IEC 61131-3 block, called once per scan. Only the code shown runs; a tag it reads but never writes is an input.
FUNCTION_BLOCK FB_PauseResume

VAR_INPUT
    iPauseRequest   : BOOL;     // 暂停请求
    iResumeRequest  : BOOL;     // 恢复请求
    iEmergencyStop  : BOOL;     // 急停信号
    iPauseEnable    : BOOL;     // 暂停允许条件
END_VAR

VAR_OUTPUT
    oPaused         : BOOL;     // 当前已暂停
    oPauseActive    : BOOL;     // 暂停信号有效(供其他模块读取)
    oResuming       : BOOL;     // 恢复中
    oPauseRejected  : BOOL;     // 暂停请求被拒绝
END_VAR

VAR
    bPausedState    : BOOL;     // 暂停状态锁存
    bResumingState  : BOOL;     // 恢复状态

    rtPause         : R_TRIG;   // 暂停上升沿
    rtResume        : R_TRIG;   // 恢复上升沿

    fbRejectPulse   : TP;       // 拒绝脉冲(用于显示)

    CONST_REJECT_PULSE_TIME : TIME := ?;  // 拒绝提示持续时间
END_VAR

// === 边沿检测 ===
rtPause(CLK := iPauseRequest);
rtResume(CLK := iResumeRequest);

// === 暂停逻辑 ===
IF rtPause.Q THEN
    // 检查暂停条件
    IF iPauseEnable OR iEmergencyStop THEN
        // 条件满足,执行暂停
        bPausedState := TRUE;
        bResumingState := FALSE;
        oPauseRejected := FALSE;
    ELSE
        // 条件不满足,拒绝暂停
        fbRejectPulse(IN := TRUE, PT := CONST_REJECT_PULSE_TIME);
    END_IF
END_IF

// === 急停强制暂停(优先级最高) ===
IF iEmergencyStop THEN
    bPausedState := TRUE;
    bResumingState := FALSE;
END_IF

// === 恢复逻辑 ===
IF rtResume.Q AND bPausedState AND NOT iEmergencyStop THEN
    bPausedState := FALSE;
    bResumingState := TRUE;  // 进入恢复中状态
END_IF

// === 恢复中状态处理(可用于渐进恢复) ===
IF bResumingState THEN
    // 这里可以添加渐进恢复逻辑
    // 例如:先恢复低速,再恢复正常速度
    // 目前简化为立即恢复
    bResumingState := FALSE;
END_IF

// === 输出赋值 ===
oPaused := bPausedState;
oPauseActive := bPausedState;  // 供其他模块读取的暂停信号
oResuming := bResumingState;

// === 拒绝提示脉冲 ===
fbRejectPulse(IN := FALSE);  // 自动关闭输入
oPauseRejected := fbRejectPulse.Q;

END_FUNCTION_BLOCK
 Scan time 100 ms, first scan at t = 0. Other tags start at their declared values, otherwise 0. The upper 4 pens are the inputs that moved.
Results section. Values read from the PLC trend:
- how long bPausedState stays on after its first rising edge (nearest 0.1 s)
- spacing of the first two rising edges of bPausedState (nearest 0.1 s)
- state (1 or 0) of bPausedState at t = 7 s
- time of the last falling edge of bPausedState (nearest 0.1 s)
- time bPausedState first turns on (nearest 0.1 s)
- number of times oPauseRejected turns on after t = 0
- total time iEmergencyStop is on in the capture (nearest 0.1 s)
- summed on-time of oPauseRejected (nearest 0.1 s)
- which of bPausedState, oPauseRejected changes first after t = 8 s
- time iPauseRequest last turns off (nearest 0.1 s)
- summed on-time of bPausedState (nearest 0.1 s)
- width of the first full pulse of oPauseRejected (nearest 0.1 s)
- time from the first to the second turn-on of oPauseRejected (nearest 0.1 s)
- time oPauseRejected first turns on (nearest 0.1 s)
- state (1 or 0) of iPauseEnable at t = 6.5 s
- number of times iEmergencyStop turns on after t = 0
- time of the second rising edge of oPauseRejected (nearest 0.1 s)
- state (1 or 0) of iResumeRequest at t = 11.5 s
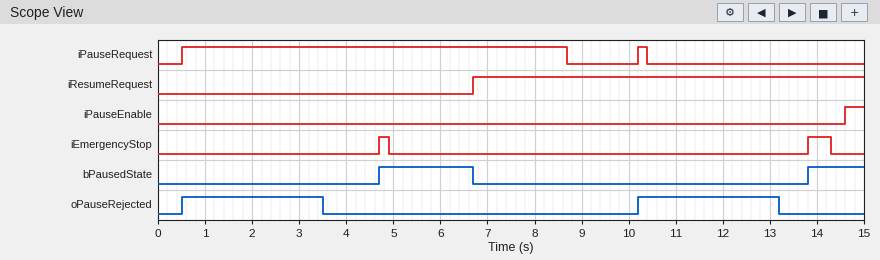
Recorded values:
2.0 s
9.1 s
0
6.7 s
4.7 s
2
0.7 s
6.0 s
oPauseRejected
10.4 s
3.2 s
3.0 s
9.7 s
0.5 s
0
2
10.2 s
1
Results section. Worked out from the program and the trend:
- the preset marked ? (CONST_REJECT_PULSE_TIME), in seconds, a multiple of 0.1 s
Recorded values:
3.0 s
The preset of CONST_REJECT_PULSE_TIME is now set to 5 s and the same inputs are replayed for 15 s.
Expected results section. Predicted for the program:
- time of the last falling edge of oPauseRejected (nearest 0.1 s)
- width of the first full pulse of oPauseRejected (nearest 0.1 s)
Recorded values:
5.5 s
5.0 s
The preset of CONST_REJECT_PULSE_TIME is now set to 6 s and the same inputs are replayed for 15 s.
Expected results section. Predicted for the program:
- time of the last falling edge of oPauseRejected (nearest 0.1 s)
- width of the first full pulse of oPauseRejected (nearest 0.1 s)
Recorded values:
6.5 s
6.0 s
